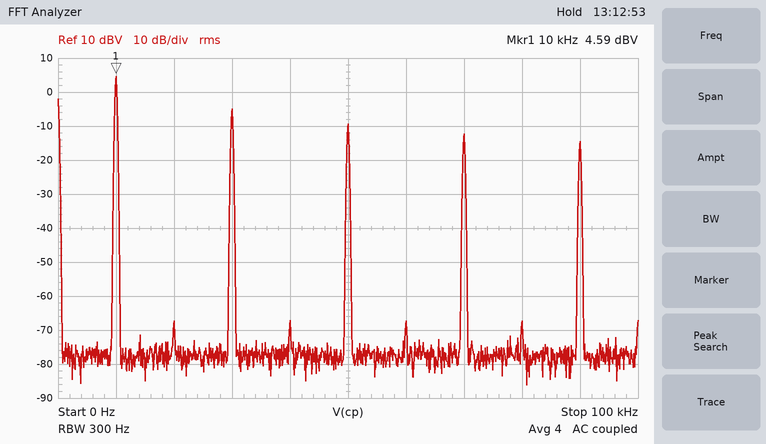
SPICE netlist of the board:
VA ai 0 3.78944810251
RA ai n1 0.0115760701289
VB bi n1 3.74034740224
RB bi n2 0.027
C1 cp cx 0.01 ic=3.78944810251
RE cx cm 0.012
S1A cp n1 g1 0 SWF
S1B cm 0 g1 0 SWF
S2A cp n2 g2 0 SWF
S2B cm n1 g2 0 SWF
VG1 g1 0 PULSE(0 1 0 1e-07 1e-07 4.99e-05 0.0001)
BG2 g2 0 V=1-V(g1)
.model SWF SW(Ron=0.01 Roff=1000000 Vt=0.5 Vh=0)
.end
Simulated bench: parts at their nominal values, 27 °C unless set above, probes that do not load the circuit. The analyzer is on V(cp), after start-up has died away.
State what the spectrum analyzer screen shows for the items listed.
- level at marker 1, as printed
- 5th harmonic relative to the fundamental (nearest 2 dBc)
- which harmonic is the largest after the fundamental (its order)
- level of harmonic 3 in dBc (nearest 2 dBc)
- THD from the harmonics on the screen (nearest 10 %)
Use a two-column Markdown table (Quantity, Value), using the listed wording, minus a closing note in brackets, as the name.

| Quantity | Value |
|---|---|
| level at marker 1, as printed | 4.59 dBV |
| 5th harmonic relative to the fundamental | -14 dBc |
| which harmonic is the largest after the fundamental | 3 |
| level of harmonic 3 in dBc | -10 dBc |
| THD from the harmonics on the screen | 40 % |
